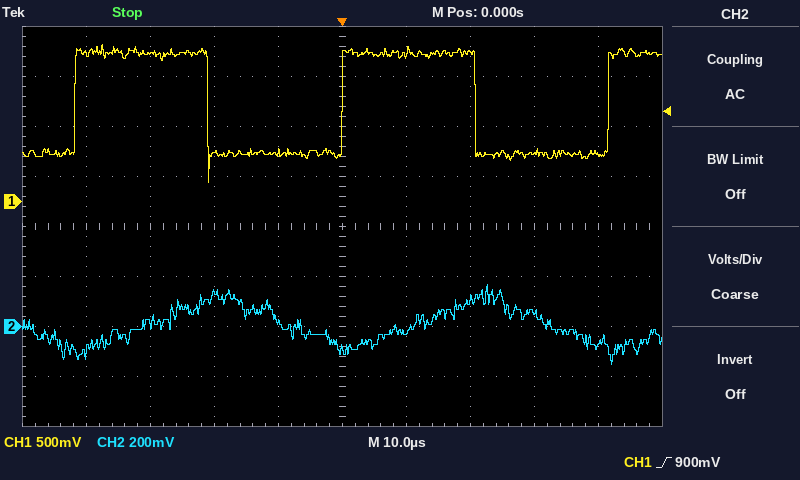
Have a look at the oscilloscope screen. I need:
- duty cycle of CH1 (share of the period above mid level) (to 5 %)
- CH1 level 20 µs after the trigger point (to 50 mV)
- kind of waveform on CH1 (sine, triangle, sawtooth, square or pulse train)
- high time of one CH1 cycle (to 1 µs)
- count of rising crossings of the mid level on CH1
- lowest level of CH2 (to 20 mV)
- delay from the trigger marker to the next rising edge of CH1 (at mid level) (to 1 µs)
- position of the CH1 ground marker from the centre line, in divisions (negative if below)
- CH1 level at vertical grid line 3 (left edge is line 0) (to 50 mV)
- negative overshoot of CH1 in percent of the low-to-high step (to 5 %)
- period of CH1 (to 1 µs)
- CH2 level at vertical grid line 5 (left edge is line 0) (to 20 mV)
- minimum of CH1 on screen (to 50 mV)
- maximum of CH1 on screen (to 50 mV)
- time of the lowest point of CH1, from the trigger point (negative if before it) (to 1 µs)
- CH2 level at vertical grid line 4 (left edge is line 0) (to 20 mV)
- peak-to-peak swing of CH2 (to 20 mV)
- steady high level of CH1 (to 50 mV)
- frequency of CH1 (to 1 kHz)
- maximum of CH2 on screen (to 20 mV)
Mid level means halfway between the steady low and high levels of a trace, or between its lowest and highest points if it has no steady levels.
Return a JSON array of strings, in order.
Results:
["50 %", "1.50 V", "square", "21 µs", "3", "-160 mV", "42 µs", "+0.5 div", "500 mV", "30 %", "42 µs", "-100 mV", "200 mV", "1.55 V", "-21 µs", "20 mV", "320 mV", "1.50 V", "24 kHz", "160 mV"]
